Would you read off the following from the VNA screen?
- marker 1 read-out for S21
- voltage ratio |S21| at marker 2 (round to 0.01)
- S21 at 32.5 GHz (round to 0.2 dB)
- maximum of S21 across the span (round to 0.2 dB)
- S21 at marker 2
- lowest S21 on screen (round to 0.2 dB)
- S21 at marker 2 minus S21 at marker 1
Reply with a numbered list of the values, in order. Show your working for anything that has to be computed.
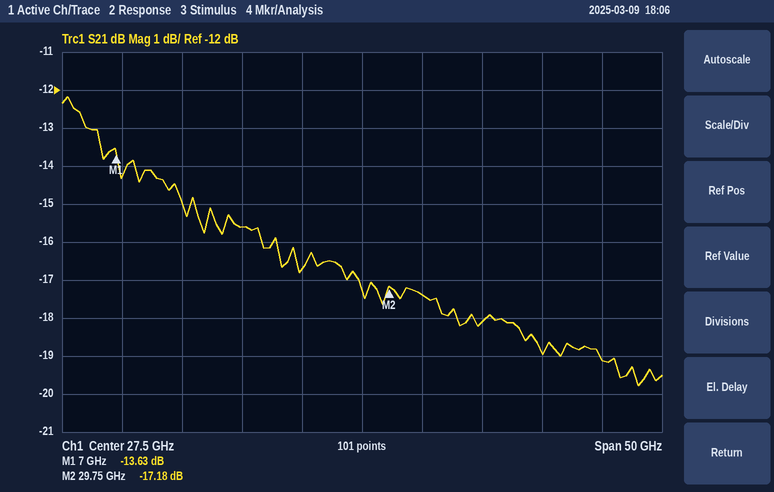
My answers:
1. -13.63 dB
2. 10^(-17.18/20) ≈ 0.14
3. -17.4 dB
4. -12.2 dB
5. -17.18 dB
6. -19.8 dB
7. -17.18 − (-13.63) = -3.55 dB
